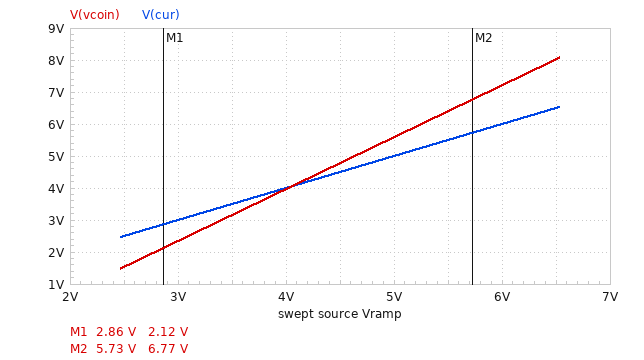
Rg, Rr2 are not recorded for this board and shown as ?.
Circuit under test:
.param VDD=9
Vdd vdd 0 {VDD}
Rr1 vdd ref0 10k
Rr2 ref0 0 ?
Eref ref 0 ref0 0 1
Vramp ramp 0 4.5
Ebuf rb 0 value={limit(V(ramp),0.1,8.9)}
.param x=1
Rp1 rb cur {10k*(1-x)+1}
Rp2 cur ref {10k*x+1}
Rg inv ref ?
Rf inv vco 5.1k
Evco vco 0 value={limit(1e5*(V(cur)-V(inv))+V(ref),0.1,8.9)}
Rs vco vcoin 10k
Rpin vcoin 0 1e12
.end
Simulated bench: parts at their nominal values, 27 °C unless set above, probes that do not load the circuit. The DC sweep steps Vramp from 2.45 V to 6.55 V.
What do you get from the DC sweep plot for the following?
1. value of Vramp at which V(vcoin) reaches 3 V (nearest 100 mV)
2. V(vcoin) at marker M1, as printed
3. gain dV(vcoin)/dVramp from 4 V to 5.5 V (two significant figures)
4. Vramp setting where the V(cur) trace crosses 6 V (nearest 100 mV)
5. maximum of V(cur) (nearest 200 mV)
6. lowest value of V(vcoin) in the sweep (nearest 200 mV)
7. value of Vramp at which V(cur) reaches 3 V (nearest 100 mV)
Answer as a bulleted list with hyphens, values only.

- 3.4 V
- 2.12 V
- 1.6 V/V
- 6.0 V
- 6.6 V
- 1.4 V
- 3.0 V
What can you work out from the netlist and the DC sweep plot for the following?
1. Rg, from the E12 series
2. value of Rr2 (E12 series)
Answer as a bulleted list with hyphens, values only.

- 8.2 kΩ
- 8.2 kΩ
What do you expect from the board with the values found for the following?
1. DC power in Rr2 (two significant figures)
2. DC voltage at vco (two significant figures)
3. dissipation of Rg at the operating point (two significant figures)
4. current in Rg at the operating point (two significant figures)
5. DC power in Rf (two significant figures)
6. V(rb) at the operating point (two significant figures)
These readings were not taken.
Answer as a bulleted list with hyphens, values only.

- 2.0 mW
- 4.8 V
- 24 µW
- 54 µA
- 15 µW
- 4.5 V
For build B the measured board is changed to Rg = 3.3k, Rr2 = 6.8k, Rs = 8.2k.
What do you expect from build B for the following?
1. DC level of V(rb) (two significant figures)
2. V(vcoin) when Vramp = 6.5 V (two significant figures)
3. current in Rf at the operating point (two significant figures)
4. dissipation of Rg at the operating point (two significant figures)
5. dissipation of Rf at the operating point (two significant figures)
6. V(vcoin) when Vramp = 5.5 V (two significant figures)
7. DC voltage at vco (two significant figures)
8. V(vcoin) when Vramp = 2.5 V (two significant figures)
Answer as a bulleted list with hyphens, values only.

- 4.5 V
- 8.9 V
- 260 µA
- 220 µW
- 340 µW
- 8.4 V
- 5.8 V
- 730 mV
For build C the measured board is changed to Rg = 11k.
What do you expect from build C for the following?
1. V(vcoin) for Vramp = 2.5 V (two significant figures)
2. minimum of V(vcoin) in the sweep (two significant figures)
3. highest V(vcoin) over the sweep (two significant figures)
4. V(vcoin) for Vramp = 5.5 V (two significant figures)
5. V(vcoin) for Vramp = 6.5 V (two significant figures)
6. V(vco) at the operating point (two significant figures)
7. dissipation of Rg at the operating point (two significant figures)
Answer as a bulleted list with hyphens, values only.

- 1.8 V
- 1.7 V
- 7.7 V
- 6.2 V
- 7.6 V
- 4.7 V
- 18 µW
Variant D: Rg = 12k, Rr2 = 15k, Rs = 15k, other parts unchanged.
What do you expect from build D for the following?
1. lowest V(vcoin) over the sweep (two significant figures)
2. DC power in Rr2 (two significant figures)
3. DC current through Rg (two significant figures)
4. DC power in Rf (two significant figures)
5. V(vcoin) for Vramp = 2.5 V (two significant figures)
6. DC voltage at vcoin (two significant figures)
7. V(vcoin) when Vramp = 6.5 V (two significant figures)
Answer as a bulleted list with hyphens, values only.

- 1.2 V
- 1.9 mW
- 75 µA
- 29 µW
- 1.3 V
- 4.1 V
- 7.0 V
